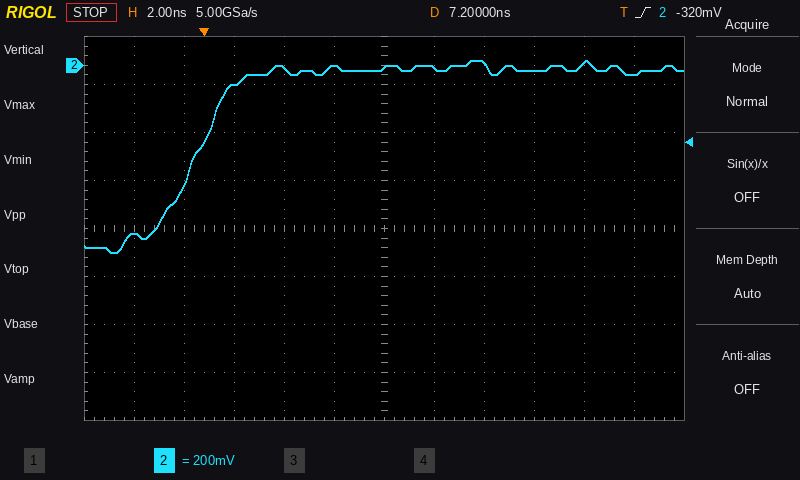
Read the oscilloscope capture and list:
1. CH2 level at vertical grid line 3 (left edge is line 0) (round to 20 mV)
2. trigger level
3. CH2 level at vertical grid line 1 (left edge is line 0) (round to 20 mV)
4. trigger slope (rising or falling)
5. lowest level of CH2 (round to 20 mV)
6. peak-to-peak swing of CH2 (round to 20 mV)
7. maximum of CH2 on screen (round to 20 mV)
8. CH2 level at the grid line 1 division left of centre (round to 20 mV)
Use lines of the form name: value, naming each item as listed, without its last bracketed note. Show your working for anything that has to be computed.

CH2 level at vertical grid line 3 (left edge is line 0): -80 mV
trigger level: -320 mV
CH2 level at vertical grid line 1 (left edge is line 0): -700 mV
trigger slope: rising
lowest level of CH2: -780 mV
peak-to-peak swing of CH2: 20 mV − (-780 mV) = 800 mV
maximum of CH2 on screen: 20 mV
CH2 level at the grid line 1 division left of centre: 0 mV
